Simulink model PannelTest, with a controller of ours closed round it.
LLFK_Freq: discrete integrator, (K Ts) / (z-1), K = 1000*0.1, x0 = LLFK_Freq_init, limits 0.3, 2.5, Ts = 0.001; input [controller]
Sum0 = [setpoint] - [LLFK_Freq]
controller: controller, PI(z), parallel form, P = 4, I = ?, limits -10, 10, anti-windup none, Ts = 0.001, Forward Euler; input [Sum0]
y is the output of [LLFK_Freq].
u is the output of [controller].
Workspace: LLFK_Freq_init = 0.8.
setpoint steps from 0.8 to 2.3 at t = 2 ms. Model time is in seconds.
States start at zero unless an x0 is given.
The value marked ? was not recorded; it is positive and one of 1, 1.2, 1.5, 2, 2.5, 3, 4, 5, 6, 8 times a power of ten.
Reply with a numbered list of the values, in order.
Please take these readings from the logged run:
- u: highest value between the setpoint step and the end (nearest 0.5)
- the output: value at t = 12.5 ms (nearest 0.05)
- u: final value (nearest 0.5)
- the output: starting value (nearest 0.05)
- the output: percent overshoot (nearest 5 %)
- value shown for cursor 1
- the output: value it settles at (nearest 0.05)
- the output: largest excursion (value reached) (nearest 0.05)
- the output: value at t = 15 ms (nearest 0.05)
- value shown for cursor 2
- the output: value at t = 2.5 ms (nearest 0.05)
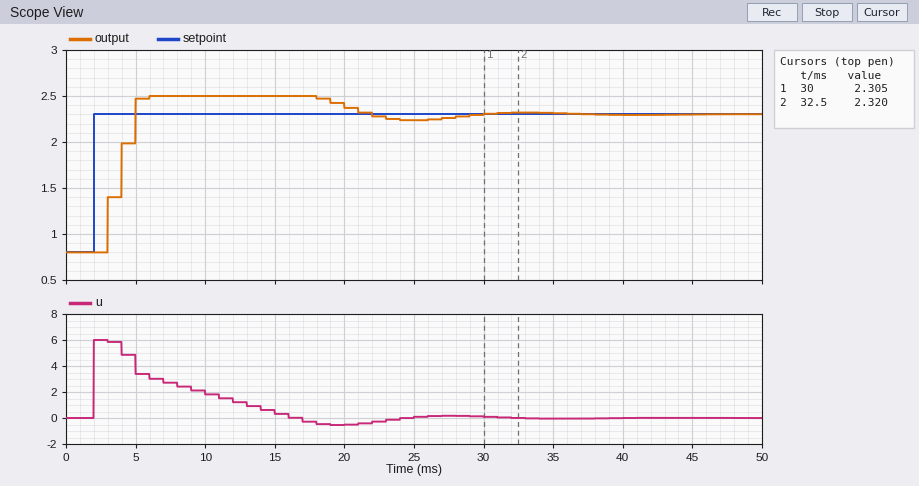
1. 6.0
2. 2.50
3. 0.0
4. 0.80
5. 15 %
6. 2.305
7. 2.30
8. 2.50
9. 2.50
10. 2.320
11. 0.80
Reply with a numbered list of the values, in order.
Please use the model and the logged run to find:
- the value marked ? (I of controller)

1. 1500
